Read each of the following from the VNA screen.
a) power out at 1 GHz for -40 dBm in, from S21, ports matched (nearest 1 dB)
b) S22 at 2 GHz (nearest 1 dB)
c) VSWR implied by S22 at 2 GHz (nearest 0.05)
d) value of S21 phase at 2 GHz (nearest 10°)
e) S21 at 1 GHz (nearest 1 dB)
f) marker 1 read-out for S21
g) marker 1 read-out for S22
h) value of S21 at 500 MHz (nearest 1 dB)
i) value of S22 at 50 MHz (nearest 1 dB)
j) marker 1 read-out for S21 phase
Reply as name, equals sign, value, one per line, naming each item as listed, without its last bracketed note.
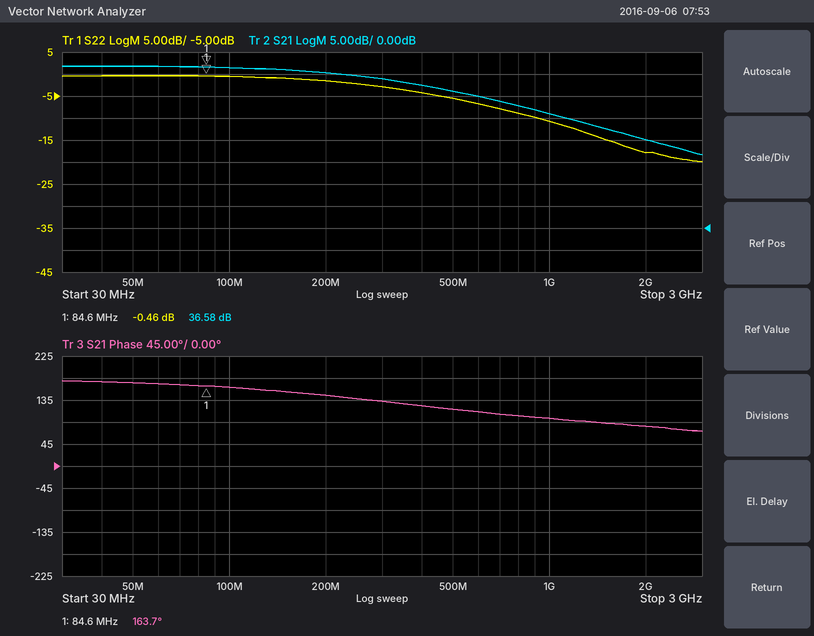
power out at 1 GHz for -40 dBm in, from S21, ports matched = -14 dBm
S22 at 2 GHz = -18 dB
VSWR implied by S22 at 2 GHz = 1.30
value of S21 phase at 2 GHz = 80°
S21 at 1 GHz = 26 dB
marker 1 read-out for S21 = 36.58 dB
marker 1 read-out for S22 = -0.46 dB
value of S21 at 500 MHz = 31 dB
value of S22 at 50 MHz = 0 dB
marker 1 read-out for S21 phase = 163.7°
